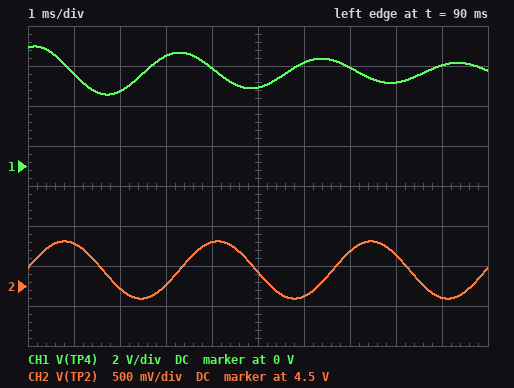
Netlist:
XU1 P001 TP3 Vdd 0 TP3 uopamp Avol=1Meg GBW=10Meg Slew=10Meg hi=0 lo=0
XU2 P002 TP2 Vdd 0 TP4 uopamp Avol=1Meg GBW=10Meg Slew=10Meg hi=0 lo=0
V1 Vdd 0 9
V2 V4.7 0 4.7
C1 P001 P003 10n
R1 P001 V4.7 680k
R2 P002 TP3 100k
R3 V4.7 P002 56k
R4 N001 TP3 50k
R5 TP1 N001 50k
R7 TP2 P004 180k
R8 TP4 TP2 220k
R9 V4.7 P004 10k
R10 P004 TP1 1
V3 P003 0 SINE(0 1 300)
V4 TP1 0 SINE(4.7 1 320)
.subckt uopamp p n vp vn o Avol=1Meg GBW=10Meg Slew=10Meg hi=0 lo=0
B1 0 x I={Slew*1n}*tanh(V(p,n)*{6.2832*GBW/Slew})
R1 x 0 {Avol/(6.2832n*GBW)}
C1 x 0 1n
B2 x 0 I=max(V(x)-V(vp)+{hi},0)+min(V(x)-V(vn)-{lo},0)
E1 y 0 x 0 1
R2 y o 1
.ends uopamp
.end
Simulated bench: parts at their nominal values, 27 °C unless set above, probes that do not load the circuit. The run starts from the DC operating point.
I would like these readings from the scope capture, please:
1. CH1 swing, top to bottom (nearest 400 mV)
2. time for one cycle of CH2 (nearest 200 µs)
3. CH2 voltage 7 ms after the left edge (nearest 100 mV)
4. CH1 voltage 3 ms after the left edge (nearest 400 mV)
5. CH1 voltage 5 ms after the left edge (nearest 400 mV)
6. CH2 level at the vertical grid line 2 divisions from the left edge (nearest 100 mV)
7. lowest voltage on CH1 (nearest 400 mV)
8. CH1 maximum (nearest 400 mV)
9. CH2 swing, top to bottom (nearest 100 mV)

2.4 V
3.4 ms
4.9 V
5.6 V
4.0 V
4.5 V
3.6 V
6.0 V
700 mV
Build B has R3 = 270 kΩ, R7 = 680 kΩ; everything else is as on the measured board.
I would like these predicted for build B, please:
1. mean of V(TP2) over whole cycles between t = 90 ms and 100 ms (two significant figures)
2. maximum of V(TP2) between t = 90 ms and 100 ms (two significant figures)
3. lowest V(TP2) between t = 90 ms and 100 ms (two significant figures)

4.7 V
5.4 V
4.0 V
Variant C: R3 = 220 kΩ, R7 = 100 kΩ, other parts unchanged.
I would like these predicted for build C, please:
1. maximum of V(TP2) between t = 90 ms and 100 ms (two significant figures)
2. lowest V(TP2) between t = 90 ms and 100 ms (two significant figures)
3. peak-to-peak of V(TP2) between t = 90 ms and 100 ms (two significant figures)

5.4 V
4.0 V
1.4 V
